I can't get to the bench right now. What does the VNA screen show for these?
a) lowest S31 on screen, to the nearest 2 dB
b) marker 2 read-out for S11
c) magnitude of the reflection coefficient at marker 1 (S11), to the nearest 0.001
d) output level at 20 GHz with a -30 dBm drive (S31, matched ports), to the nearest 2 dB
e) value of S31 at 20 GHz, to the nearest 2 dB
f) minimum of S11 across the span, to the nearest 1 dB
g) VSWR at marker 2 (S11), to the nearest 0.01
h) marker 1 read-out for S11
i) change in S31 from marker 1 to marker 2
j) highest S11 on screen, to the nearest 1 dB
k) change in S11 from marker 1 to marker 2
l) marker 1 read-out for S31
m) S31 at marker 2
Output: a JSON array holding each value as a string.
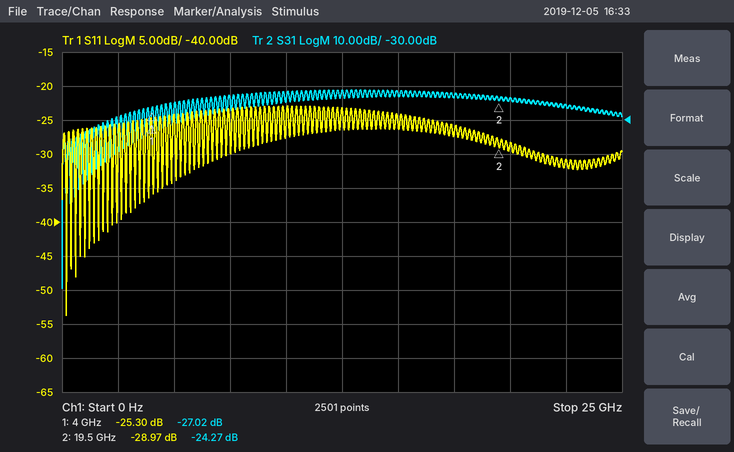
["-80 dB", "-28.97 dB", "0.054", "-54 dBm", "-24 dB", "-54 dB", "1.07", "-25.30 dB", "2.75 dB", "-23 dB", "-3.67 dB", "-27.02 dB", "-24.27 dB"]
